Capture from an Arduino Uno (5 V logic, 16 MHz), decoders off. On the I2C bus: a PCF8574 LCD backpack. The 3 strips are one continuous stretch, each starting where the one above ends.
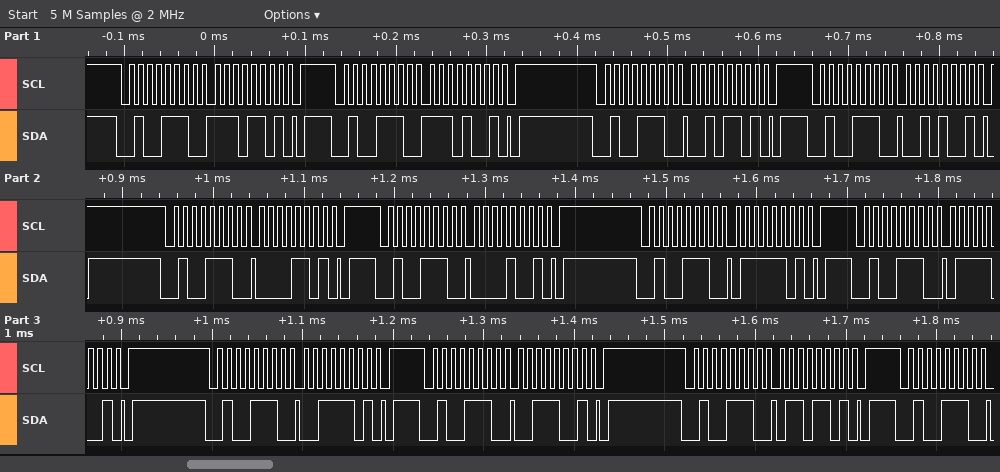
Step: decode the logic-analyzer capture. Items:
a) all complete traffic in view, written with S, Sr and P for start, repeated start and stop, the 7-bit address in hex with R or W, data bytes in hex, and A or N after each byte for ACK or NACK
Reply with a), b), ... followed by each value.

a) S 27W A ED A P S 27W A E9 A P S 27W A 2D A P S 27W A 29 A P S 27W A 0D A P S 27W A 09 A P S 27W A 7D A P S 27W A 79 A P S 27W A 3D A P S 27W A 39 A P S 27W A 6D A P S 27W A
